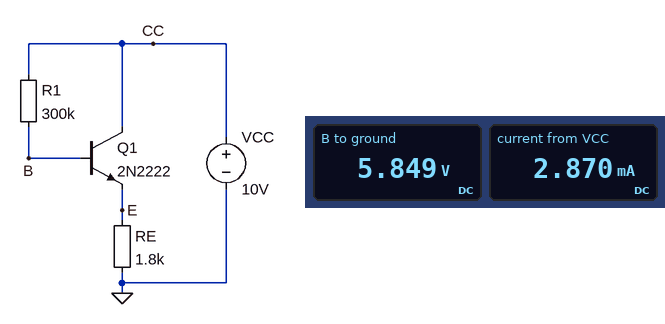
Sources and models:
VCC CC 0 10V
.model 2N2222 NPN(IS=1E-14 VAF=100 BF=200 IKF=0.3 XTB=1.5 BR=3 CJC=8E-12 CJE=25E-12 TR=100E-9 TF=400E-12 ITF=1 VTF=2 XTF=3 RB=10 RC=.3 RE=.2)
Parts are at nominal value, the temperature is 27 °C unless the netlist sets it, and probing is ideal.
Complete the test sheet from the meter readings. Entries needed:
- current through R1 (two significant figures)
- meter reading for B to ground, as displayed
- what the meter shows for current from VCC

14 µA
5.849 V
2.870 mA
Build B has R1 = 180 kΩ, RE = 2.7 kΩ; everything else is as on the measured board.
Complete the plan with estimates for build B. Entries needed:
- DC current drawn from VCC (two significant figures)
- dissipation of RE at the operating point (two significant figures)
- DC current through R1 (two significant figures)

2.6 mA
18 mW
13 µA
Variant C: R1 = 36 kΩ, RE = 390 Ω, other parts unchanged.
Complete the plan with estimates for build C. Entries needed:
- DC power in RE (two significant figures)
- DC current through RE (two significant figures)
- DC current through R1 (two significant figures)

100 mW
16 mA
82 µA
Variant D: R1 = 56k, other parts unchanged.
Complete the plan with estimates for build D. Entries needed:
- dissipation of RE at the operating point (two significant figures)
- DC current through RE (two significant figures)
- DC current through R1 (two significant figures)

36 mW
4.5 mA
22 µA
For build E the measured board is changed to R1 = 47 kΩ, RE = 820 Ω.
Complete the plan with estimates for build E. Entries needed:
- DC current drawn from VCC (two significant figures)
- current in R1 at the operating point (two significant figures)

8.8 mA
44 µA
